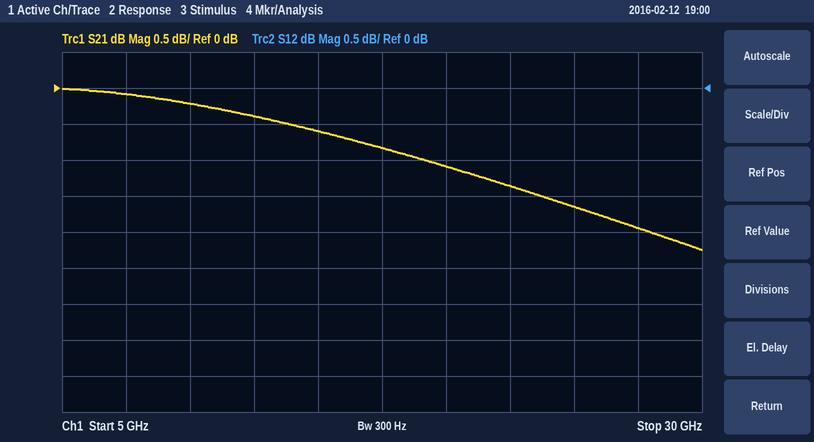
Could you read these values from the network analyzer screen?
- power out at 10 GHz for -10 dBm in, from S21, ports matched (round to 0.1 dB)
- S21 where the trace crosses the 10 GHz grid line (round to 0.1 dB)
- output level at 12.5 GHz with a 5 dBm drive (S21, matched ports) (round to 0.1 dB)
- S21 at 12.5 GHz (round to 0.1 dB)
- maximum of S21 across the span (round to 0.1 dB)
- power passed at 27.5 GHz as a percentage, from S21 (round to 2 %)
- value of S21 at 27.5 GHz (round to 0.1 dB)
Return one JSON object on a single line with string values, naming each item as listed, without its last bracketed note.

{"power out at 10 GHz for -10 dBm in, from S21, ports matched": "-10.2 dBm", "S21 where the trace crosses the 10 GHz grid line": "-0.2 dB", "output level at 12.5 GHz with a 5 dBm drive (S21, matched ports)": "4.6 dBm", "S21 at 12.5 GHz": "-0.4 dB", "maximum of S21 across the span": "0.0 dB", "power passed at 27.5 GHz as a percentage, from S21": "64 %", "value of S21 at 27.5 GHz": "-1.9 dB"}
